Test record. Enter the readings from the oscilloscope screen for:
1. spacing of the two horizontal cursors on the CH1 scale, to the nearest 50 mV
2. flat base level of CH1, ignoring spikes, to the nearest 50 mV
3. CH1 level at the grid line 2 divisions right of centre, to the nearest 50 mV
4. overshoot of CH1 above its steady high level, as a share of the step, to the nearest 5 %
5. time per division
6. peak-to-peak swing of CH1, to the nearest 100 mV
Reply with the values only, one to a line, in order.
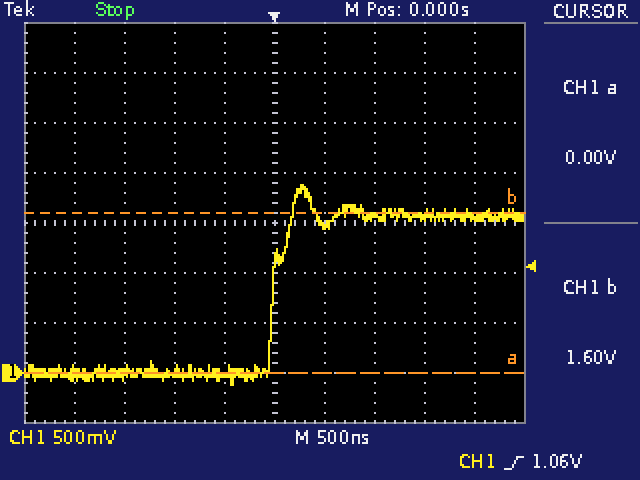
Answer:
1.60 V
0 mV
1.55 V
20 %
500 ns
2.00 V
